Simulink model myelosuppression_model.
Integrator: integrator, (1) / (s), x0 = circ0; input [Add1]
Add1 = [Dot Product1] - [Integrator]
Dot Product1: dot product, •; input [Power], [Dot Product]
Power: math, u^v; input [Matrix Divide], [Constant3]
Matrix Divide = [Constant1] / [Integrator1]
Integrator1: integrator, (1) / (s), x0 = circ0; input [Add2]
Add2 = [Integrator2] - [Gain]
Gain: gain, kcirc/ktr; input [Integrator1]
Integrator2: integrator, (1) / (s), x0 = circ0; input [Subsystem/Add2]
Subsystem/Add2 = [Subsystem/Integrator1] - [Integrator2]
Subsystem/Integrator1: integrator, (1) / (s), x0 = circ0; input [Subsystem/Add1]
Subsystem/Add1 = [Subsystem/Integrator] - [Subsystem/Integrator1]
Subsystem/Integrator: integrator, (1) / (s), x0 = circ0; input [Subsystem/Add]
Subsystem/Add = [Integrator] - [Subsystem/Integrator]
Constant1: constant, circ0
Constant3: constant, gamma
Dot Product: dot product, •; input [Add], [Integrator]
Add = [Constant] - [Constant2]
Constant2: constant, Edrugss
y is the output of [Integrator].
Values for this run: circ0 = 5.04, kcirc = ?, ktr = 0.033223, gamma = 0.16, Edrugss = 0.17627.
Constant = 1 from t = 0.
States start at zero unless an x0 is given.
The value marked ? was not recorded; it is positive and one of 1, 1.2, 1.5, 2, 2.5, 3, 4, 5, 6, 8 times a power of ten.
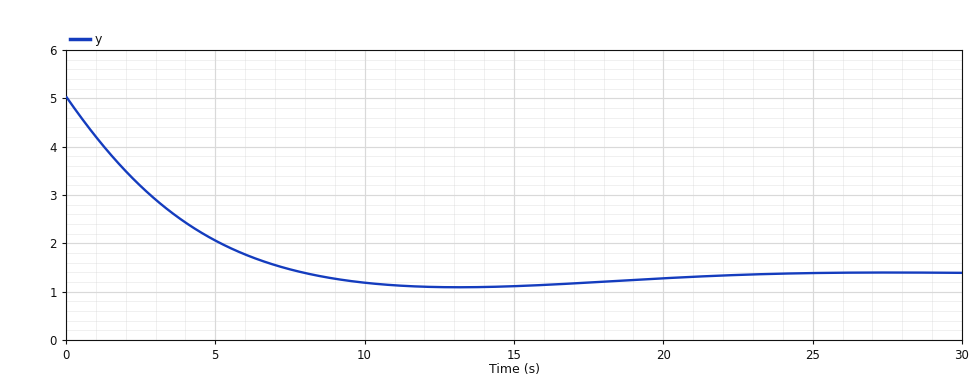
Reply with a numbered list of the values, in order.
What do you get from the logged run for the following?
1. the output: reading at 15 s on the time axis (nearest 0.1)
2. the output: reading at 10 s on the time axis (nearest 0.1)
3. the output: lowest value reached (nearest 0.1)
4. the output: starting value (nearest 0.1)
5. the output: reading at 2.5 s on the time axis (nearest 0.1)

1. 1.1
2. 1.2
3. 1.1
4. 5.0
5. 3.2
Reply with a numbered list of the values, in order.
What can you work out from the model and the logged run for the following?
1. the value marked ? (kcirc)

1. 0.03
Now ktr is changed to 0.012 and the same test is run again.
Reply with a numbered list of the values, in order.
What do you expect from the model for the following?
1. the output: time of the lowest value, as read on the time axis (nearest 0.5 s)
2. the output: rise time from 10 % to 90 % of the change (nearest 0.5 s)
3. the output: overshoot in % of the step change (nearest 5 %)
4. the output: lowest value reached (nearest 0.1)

1. 10.5 s
2. 4.5 s
3. 10 %
4. 3.6
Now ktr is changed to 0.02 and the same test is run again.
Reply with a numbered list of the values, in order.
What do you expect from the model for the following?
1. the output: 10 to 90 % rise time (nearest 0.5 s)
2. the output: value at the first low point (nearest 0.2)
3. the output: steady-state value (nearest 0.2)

1. 5.5 s
2. 2.0
3. 2.2
